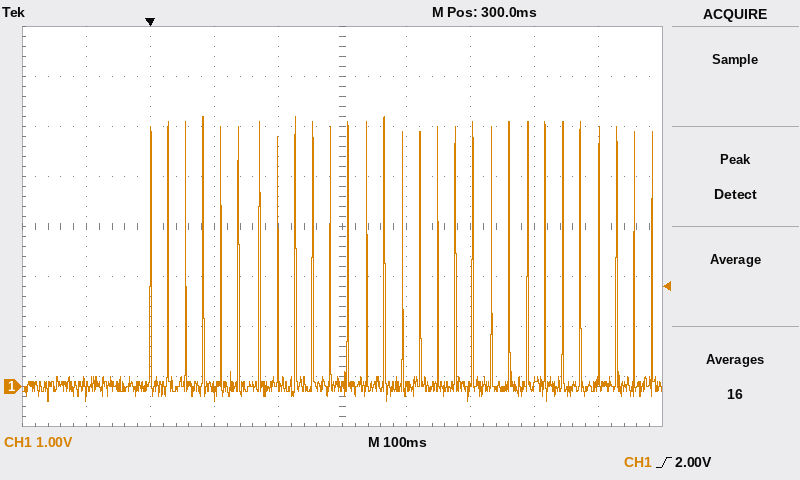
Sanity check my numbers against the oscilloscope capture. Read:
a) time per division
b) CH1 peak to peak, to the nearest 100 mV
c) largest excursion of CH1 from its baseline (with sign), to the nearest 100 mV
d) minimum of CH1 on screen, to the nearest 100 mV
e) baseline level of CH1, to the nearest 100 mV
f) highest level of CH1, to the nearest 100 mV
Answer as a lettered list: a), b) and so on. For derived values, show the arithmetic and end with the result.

a) 100 ms
b) 5.4 V − (-300 mV) = 5.7 V
c) 5.4 V − (0.0 V) = +5.4 V
d) -300 mV
e) 0.0 V
f) 5.4 V
